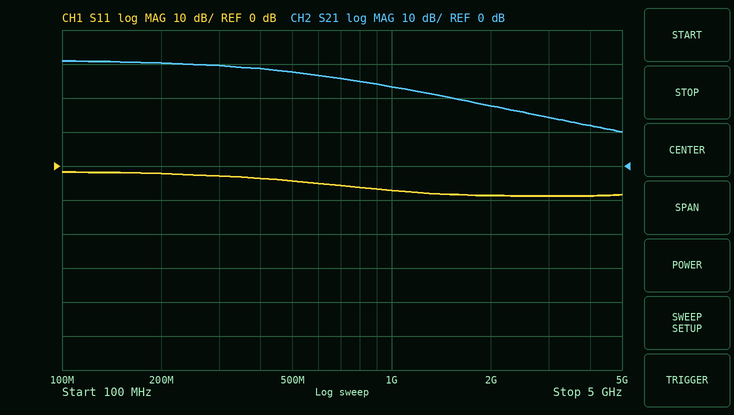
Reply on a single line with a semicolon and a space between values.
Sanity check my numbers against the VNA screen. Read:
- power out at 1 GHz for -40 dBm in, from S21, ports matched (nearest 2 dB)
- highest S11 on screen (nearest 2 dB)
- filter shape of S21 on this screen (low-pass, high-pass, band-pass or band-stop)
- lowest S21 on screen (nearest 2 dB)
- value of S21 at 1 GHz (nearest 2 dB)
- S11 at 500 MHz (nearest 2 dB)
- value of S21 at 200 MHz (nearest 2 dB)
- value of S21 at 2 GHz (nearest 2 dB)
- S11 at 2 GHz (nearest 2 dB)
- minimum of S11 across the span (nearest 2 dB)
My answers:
-16 dBm; -2 dB; low-pass; 10 dB; 24 dB; -4 dB; 30 dB; 18 dB; -8 dB; -8 dB
